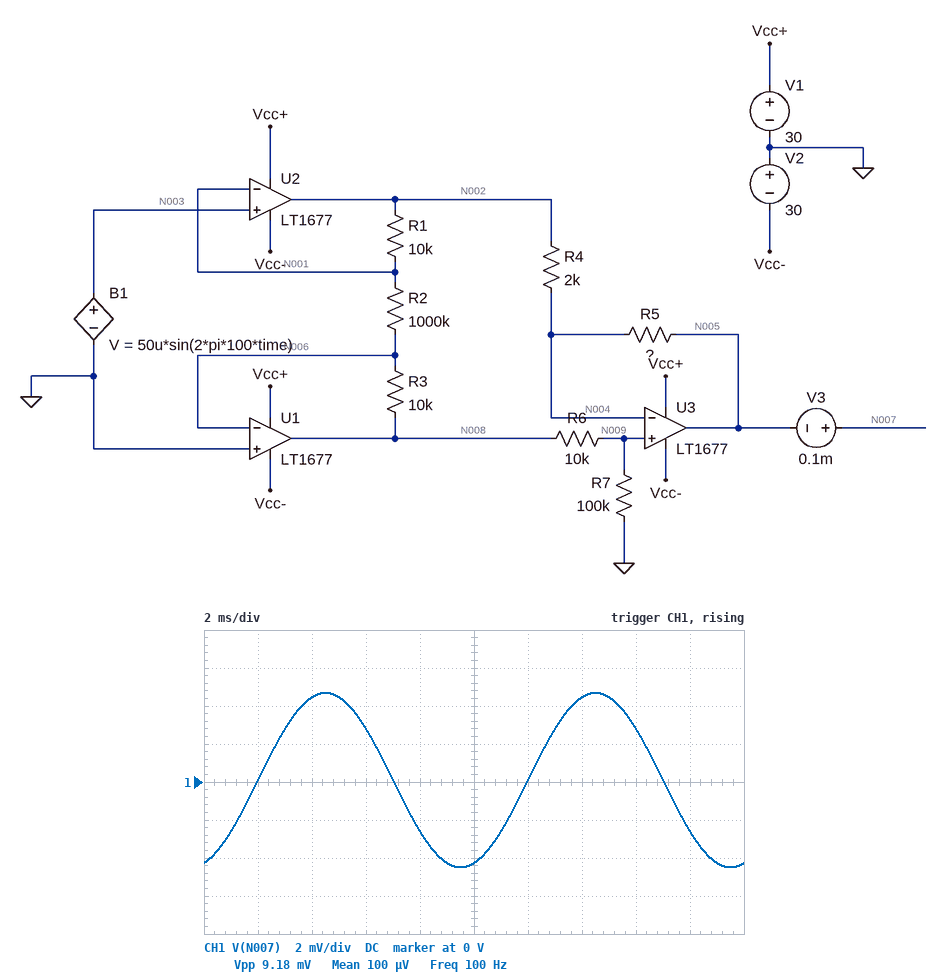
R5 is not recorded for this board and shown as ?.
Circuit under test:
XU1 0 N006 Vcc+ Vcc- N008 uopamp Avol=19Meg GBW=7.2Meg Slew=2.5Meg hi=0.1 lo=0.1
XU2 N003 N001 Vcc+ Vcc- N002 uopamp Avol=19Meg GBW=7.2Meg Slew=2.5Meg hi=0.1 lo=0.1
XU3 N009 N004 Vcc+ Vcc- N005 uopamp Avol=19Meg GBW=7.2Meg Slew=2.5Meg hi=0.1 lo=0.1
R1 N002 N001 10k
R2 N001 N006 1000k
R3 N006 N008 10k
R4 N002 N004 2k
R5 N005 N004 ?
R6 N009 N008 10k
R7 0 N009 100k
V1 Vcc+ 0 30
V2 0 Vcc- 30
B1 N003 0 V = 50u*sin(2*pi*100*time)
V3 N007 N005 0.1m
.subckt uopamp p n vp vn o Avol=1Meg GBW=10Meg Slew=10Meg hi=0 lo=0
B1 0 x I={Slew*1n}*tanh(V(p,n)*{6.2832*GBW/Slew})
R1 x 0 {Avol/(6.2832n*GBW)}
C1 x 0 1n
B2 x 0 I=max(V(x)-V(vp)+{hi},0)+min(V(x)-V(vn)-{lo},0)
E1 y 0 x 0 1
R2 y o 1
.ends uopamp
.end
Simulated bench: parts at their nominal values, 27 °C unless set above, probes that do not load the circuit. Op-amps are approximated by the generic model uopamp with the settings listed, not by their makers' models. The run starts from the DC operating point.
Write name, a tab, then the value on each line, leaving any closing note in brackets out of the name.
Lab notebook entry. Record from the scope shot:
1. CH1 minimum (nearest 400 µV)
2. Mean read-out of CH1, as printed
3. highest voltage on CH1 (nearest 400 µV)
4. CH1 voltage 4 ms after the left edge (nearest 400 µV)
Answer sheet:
CH1 minimum	-4.4 mV
Mean read-out of CH1, as printed	100 µV
highest voltage on CH1	4.8 mV
CH1 voltage 4 ms after the left edge	4.4 mV
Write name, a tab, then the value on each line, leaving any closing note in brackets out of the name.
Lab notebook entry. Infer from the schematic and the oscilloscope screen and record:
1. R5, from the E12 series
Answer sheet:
R5, from the E12 series	180 kΩ
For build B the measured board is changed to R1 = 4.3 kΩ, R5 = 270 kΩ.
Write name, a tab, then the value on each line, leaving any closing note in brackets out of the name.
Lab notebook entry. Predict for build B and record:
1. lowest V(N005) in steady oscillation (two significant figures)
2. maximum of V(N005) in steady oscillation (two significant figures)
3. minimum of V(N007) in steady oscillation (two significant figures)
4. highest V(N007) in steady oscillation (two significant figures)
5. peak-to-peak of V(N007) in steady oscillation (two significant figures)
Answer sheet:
lowest V(N005) in steady oscillation	-6.8 mV
maximum of V(N005) in steady oscillation	6.8 mV
minimum of V(N007) in steady oscillation	-6.7 mV
highest V(N007) in steady oscillation	6.9 mV
peak-to-peak of V(N007) in steady oscillation	14 mV
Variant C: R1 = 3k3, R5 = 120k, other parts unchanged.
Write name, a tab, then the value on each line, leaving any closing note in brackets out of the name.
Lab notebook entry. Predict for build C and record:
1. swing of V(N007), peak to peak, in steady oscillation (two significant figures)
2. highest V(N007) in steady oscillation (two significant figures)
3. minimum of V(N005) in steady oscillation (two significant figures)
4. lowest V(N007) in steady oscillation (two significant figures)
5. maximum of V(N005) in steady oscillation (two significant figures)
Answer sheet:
swing of V(N007), peak to peak, in steady oscillation	6.1 mV
highest V(N007) in steady oscillation	3.1 mV
minimum of V(N005) in steady oscillation	-3.0 mV
lowest V(N007) in steady oscillation	-2.9 mV
maximum of V(N005) in steady oscillation	3.0 mV
